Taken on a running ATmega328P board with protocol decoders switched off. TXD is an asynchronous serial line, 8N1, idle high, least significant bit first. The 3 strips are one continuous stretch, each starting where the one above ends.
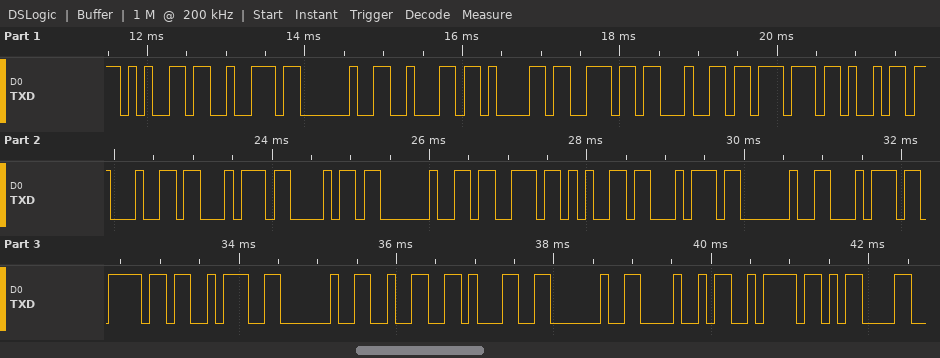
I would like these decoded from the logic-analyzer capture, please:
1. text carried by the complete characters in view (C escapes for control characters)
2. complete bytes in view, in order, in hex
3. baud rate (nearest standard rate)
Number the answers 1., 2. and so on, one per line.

1. "er bandwidth set to: 21 Hz\r"
2. 65 72 20 62 61 6E 64 77 69 64 74 68 20 73 65 74 20 74 6F 3A 20 32 31 20 48 7A 0D
3. 9600 baud
